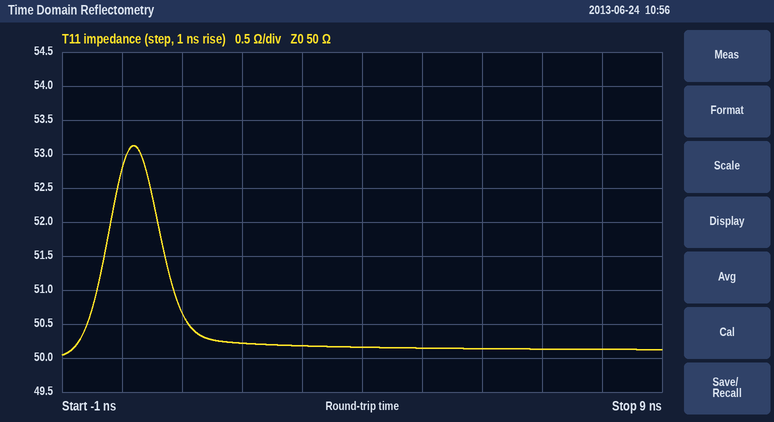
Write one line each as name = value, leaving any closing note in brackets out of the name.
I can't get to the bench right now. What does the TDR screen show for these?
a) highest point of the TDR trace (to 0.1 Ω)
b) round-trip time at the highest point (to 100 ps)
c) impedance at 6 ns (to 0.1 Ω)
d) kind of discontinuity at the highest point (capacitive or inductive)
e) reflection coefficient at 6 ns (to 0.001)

highest point of the TDR trace = 53.1 Ω
round-trip time at the highest point = 200 ps
impedance at 6 ns = 50.1 Ω
kind of discontinuity at the highest point = inductive
reflection coefficient at 6 ns = +0.001
